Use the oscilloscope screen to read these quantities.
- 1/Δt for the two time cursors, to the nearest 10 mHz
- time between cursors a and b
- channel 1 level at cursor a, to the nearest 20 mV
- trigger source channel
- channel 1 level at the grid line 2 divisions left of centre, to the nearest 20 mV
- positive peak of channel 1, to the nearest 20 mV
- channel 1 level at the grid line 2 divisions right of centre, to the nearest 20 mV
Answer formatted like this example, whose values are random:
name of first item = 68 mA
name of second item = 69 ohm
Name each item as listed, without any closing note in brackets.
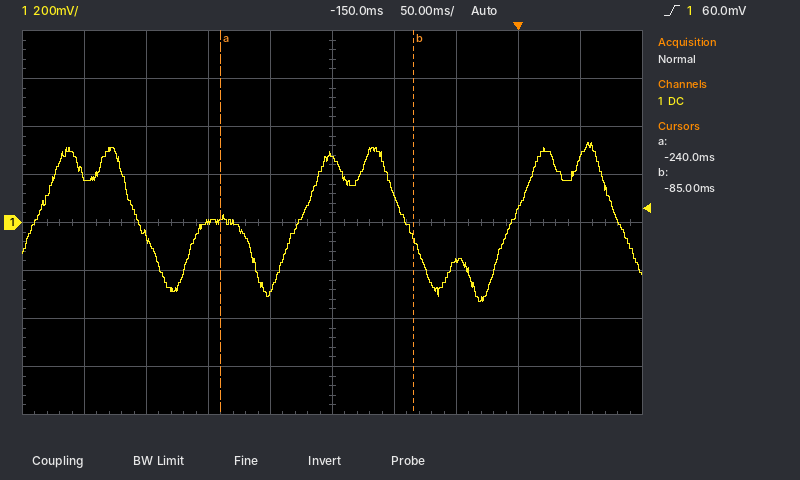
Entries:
1/Δt for the two time cursors, to the nearest 10 mHz = 6.45 Hz
time between cursors a and b = 155 ms
channel 1 level at cursor a, to the nearest 20 mV = 20 mV
trigger source channel = channel 1
channel 1 level at the grid line 2 divisions left of centre, to the nearest 20 mV = 0 mV
positive peak of channel 1, to the nearest 20 mV = 340 mV
channel 1 level at the grid line 2 divisions right of centre, to the nearest 20 mV = -160 mV
